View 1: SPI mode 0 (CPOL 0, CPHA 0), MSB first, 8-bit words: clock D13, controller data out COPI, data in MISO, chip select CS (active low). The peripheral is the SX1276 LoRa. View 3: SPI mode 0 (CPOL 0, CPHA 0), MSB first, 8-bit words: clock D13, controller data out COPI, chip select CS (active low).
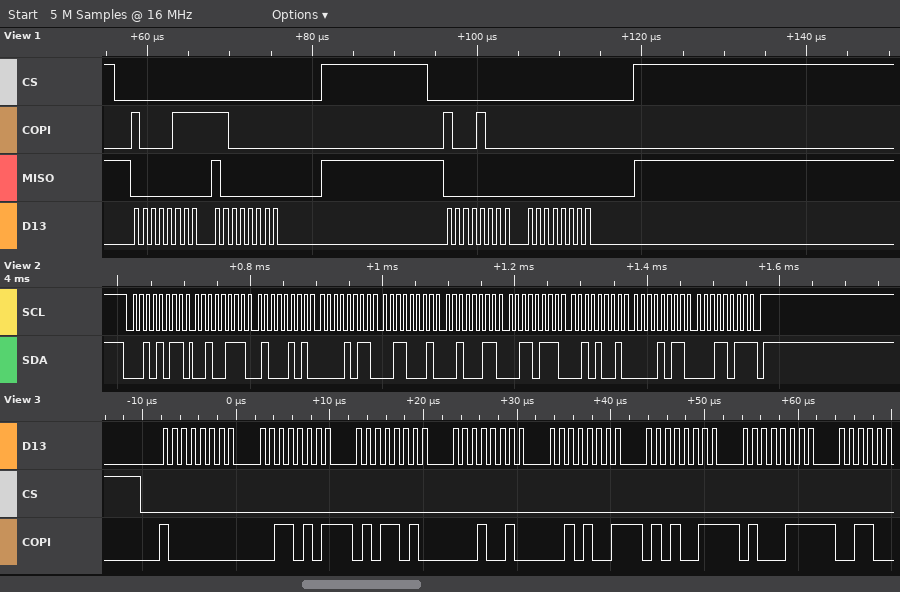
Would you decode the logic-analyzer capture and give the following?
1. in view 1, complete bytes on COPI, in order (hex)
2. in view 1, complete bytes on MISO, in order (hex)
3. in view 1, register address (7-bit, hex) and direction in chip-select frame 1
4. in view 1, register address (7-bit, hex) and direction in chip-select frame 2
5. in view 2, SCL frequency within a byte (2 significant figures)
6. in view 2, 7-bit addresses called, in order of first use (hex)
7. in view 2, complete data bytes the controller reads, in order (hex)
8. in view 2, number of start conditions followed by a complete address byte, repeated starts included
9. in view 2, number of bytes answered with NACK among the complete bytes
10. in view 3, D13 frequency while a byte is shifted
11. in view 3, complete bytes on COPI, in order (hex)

0x87 0xC0 0x88 0x00
0x00 0x80 0x00 0x00
0x07 write
0x08 write
100 kHz
0x15
27 45 0B 31 23 37 29 0B 1B
1
1
1 MHz
80 35 5A 12 29 53 47
